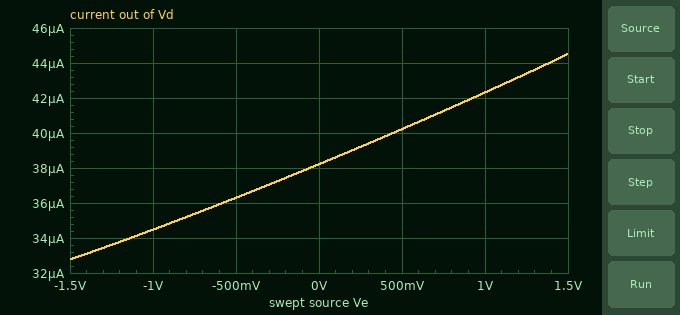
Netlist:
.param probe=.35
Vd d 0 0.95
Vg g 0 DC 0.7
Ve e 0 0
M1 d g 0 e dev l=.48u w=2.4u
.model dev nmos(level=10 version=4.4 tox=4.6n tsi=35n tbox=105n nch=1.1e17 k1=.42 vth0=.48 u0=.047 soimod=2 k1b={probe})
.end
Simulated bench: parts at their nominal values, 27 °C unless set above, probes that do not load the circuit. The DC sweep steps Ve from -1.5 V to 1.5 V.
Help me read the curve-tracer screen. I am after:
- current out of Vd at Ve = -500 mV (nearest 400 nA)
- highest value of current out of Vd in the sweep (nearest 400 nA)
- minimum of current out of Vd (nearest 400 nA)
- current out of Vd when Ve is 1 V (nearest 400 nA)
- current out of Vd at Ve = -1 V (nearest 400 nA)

36.4 µA
44.4 µA
32.8 µA
42.4 µA
34.4 µA
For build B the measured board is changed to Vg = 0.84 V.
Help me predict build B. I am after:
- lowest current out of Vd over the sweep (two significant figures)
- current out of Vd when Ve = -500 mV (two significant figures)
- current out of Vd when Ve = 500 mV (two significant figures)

60 µA
65 µA
70 µA
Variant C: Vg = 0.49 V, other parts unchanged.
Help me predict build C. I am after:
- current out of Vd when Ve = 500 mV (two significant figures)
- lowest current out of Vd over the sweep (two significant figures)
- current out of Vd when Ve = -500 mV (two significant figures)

7.8 µA
4.7 µA
6.1 µA
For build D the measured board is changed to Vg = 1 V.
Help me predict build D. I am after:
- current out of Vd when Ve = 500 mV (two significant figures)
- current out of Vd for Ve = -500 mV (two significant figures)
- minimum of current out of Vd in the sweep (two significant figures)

110 µA
100 µA
97 µA
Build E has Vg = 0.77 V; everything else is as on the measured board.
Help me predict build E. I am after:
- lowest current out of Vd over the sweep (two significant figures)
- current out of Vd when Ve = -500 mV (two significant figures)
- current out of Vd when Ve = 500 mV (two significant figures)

46 µA
50 µA
54 µA
